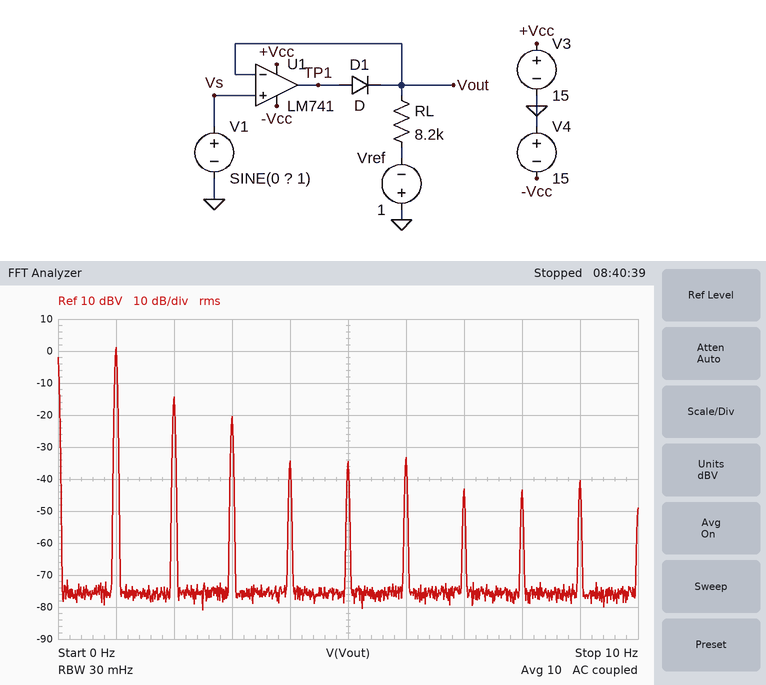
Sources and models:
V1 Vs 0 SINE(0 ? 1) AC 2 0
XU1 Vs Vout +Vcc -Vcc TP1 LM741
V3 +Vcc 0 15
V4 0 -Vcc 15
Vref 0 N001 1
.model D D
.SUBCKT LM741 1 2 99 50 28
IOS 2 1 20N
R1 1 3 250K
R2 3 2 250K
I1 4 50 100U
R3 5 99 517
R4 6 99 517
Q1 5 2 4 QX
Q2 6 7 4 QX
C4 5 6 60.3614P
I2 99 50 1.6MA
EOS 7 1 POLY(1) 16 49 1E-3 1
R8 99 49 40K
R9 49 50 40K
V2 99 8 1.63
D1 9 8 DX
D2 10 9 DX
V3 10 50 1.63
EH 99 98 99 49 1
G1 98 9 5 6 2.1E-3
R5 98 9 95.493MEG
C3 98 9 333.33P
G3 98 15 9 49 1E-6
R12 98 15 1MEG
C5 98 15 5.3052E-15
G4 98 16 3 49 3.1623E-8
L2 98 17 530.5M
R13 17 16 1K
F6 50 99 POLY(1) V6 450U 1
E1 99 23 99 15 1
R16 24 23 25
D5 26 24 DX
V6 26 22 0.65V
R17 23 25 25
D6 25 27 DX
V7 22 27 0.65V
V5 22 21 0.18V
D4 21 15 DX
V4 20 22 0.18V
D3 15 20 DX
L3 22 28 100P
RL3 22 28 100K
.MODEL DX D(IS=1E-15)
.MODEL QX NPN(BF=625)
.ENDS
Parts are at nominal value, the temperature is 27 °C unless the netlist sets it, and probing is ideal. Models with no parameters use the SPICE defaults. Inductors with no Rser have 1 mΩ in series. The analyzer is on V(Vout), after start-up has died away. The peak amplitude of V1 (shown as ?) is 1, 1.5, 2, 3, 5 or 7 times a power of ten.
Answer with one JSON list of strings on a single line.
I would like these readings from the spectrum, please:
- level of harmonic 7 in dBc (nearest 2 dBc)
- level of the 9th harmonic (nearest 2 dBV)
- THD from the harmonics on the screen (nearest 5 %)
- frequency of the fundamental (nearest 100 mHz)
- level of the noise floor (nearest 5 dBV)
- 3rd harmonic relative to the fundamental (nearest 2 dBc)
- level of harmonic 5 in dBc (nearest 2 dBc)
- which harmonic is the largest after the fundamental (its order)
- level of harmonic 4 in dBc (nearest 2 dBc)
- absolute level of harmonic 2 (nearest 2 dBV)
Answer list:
["-44 dBc", "-40 dBV", "20 %", "1.0 Hz", "-75 dBV", "-22 dBc", "-36 dBc", "2", "-36 dBc", "-14 dBV"]
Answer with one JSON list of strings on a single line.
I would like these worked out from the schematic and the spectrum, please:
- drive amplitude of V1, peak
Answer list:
["2 V"]
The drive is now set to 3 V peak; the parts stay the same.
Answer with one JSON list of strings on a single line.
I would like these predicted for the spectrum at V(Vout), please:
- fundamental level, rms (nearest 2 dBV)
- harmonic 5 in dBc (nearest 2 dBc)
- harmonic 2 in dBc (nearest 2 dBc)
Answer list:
["4 dBV", "-30 dBc", "-12 dBc"]
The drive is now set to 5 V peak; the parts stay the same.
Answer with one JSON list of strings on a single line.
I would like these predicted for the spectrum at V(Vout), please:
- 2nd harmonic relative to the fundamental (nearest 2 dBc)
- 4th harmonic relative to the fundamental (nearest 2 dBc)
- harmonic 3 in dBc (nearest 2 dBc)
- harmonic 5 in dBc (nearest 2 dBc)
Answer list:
["-10 dBc", "-26 dBc", "-24 dBc", "-30 dBc"]
